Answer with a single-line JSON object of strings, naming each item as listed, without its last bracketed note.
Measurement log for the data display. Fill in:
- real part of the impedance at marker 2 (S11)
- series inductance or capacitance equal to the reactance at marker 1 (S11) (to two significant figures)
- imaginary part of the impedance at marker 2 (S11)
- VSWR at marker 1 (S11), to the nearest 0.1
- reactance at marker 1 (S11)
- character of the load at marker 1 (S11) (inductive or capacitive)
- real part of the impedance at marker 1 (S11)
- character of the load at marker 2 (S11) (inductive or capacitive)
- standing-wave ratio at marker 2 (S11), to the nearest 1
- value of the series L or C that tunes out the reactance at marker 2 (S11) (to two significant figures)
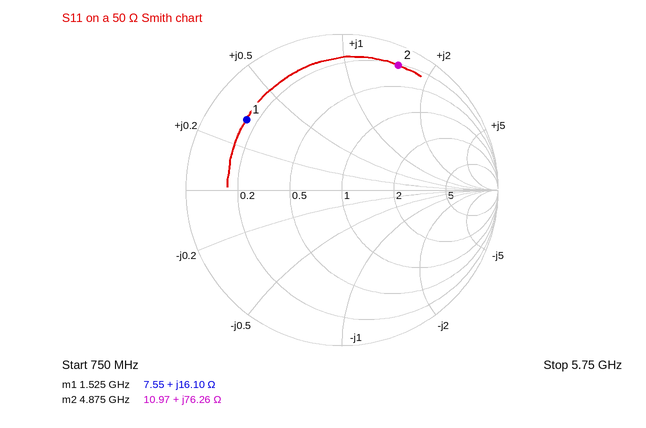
{"real part of the impedance at marker 2": "10.97 Ω", "series inductance or capacitance equal to the reactance at marker 1 (S11)": "1.7 nH", "imaginary part of the impedance at marker 2": "+76.26 Ω", "VSWR at marker 1 (S11), to the nearest 0.1": "7.3", "reactance at marker 1": "+16.10 Ω", "character of the load at marker 1 (S11)": "inductive", "real part of the impedance at marker 1": "7.55 Ω", "character of the load at marker 2 (S11)": "inductive", "standing-wave ratio at marker 2 (S11), to the nearest 1": "15", "value of the series L or C that tunes out the reactance at marker 2 (S11)": "430 fF"}
